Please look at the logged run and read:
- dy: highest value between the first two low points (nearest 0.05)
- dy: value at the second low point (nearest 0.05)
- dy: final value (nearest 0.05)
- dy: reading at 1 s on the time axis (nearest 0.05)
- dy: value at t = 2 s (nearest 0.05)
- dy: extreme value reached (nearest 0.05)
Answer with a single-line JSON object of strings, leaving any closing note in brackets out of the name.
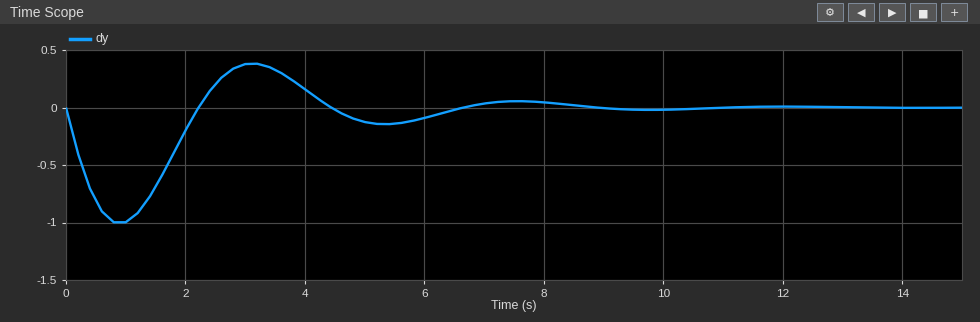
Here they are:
{"dy: highest value between the first two low points": "0.40", "dy: value at the second low point": "-0.15", "dy: final value": "0.00", "dy: reading at 1 s on the time axis": "-1.00", "dy: value at t = 2 s": "-0.20", "dy: extreme value reached": "-1.00"}
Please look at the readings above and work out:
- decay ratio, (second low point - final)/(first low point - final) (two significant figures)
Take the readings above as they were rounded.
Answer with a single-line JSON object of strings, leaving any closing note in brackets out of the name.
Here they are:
{"decay ratio, (second low point - final)/(first low point - final)": "0.15"}
